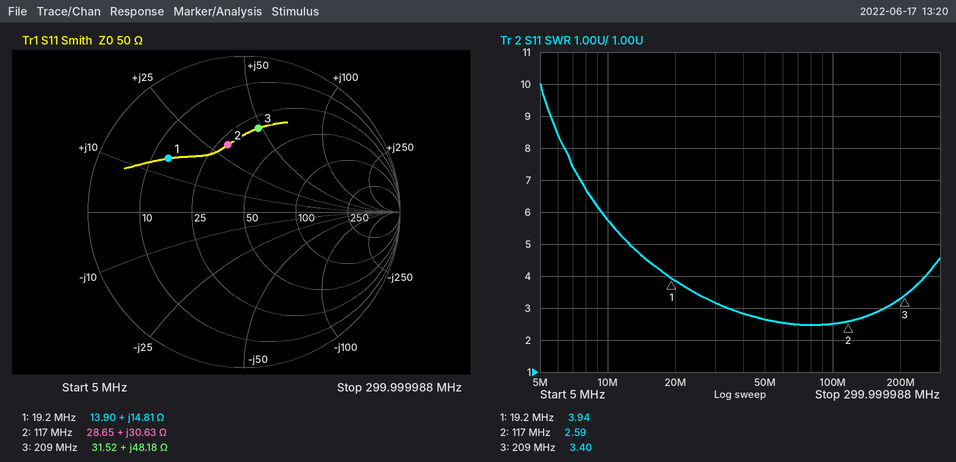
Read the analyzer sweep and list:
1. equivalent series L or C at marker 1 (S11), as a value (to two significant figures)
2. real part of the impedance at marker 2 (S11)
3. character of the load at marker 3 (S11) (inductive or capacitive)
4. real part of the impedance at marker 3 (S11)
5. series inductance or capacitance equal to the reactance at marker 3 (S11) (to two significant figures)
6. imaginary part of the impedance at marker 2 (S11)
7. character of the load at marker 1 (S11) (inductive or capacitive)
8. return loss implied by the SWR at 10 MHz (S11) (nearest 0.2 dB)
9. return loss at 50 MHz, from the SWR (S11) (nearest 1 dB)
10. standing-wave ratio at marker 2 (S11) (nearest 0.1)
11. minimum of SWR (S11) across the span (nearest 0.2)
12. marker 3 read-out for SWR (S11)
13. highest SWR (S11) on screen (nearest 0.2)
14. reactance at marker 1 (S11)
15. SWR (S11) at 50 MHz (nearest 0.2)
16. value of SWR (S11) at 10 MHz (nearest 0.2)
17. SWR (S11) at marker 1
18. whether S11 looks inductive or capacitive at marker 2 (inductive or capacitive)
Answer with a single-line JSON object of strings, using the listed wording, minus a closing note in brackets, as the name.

{"equivalent series L or C at marker 1 (S11), as a value": "120 nH", "real part of the impedance at marker 2": "28.65 Ω", "character of the load at marker 3 (S11)": "inductive", "real part of the impedance at marker 3": "31.52 Ω", "series inductance or capacitance equal to the reactance at marker 3 (S11)": "37 nH", "imaginary part of the impedance at marker 2": "+30.63 Ω", "character of the load at marker 1 (S11)": "inductive", "return loss implied by the SWR at 10 MHz (S11)": "3.0 dB", "return loss at 50 MHz, from the SWR (S11)": "7 dB", "standing-wave ratio at marker 2 (S11)": "2.6", "minimum of SWR (S11) across the span": "2.4", "marker 3 read-out for SWR": "3.40", "highest SWR (S11) on screen": "10.0", "reactance at marker 1": "+14.81 Ω", "SWR (S11) at 50 MHz": "2.6", "value of SWR (S11) at 10 MHz": "5.8", "SWR (S11) at marker 1": "3.94", "whether S11 looks inductive or capacitive at marker 2": "inductive"}
